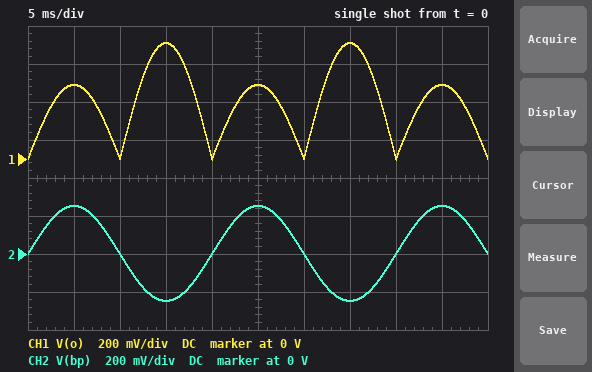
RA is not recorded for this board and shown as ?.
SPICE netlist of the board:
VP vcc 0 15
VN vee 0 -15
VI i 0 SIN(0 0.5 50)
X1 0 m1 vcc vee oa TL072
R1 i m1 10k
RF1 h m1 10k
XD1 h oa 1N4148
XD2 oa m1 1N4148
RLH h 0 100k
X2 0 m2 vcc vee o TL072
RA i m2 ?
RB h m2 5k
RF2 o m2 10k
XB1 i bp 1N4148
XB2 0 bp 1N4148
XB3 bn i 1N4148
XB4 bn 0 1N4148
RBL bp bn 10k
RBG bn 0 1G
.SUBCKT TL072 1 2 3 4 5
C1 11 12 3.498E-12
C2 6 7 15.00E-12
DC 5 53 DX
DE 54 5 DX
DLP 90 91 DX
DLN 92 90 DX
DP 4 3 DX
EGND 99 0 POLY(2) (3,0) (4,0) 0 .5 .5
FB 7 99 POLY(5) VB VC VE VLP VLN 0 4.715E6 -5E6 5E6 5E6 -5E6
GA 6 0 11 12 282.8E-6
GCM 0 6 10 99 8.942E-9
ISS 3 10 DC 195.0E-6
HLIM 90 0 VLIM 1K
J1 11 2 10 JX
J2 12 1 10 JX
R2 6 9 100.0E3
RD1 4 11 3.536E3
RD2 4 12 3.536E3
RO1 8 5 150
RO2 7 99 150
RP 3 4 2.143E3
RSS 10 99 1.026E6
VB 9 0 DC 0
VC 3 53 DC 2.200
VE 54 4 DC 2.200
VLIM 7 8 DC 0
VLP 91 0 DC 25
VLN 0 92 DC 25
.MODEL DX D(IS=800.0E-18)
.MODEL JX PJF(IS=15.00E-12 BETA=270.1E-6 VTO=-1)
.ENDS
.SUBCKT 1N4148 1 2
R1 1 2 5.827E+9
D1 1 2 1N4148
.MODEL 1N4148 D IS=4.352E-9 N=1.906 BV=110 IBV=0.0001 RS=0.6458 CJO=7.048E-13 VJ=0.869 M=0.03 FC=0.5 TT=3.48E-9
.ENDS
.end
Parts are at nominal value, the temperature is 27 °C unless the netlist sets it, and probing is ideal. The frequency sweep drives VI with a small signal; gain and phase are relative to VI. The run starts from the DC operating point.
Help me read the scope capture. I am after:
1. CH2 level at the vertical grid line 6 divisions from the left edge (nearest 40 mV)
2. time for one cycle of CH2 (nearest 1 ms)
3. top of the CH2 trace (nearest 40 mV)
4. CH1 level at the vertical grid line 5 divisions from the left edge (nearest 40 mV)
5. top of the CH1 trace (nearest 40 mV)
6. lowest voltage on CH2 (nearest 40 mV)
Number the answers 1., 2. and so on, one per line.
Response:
1. 0 V
2. 20 ms
3. 240 mV
4. 400 mV
5. 600 mV
6. -240 mV
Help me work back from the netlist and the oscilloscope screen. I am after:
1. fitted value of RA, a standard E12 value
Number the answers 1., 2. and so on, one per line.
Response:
1. 8.2 kΩ
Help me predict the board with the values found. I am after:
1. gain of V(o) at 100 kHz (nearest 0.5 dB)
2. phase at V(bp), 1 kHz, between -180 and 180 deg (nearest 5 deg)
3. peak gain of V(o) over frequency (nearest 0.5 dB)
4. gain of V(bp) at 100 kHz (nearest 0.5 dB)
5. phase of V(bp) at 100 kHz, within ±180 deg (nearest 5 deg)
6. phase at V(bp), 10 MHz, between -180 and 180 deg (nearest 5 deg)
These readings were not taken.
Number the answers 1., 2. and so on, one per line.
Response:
1. 3.5 dB
2. 0 deg
3. 3.5 dB
4. -6.0 dB
5. 0 deg
6. 0 deg
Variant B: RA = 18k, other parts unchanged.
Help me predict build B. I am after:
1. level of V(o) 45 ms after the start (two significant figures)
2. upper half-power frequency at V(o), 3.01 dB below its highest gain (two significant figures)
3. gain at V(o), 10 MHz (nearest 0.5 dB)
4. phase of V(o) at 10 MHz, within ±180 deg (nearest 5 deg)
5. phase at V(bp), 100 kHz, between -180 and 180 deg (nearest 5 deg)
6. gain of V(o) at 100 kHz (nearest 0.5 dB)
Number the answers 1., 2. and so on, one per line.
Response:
1. 720 mV
2. 2.2 MHz
3. -21.0 dB
4. 20 deg
5. 0 deg
6. -1.5 dB
